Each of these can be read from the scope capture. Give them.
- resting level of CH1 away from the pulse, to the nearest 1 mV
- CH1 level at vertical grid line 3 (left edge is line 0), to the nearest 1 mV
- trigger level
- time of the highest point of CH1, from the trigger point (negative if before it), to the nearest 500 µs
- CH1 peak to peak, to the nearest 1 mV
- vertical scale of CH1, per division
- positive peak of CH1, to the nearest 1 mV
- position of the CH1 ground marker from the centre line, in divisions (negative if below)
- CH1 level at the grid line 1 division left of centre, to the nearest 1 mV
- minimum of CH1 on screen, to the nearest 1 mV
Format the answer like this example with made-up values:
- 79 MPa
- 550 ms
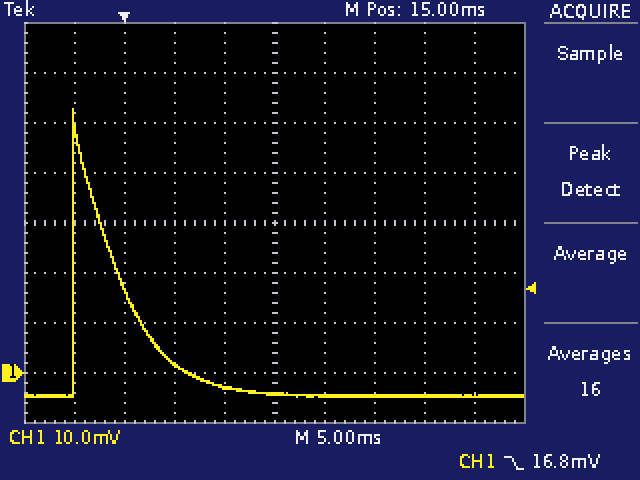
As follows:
- -5 mV
- 2 mV
- 16.8 mV
- -5.0 ms
- 58 mV
- 10 mV
- 53 mV
- -3.0 div
- -3 mV
- -5 mV
